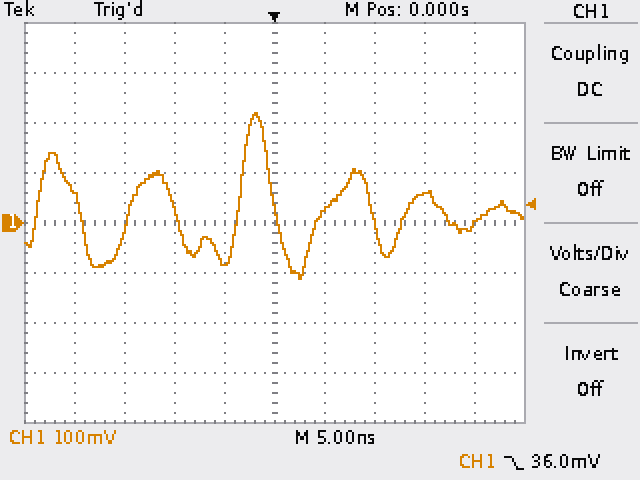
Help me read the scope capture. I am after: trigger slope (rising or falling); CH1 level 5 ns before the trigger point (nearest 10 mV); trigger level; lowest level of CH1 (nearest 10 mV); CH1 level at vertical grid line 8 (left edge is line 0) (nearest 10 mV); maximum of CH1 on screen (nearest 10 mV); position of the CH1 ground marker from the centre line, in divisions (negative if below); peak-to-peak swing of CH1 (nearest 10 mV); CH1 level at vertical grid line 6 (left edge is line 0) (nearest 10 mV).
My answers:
falling
-80 mV
36.0 mV
-110 mV
60 mV
220 mV
0.0 div
330 mV
20 mV
